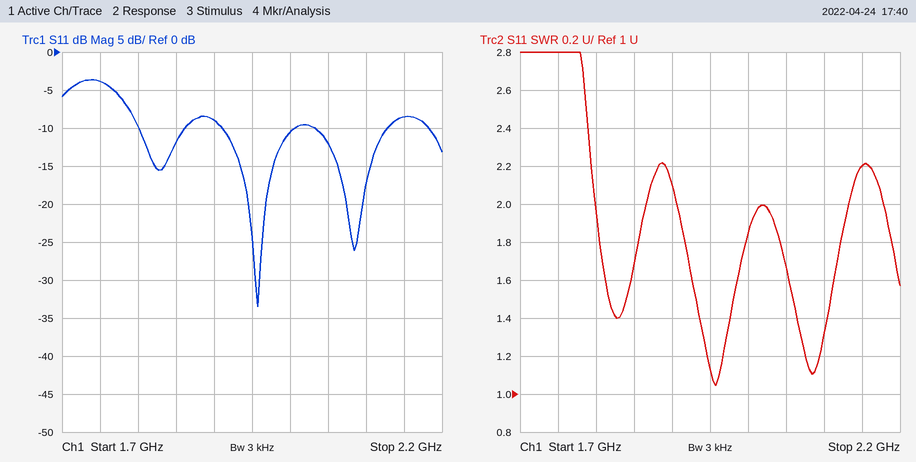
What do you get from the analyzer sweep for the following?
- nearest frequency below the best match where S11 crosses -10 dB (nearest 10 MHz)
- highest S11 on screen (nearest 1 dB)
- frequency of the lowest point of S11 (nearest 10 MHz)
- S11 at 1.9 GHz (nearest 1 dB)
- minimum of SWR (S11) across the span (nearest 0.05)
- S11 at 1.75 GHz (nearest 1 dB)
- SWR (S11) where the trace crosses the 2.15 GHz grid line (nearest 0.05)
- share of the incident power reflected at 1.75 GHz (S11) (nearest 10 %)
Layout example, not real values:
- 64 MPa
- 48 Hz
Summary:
- 1.91 GHz
- -4 dB
- 1.96 GHz
- -9 dB
- 1.05
- -4 dB
- 2.20
- 40 %
